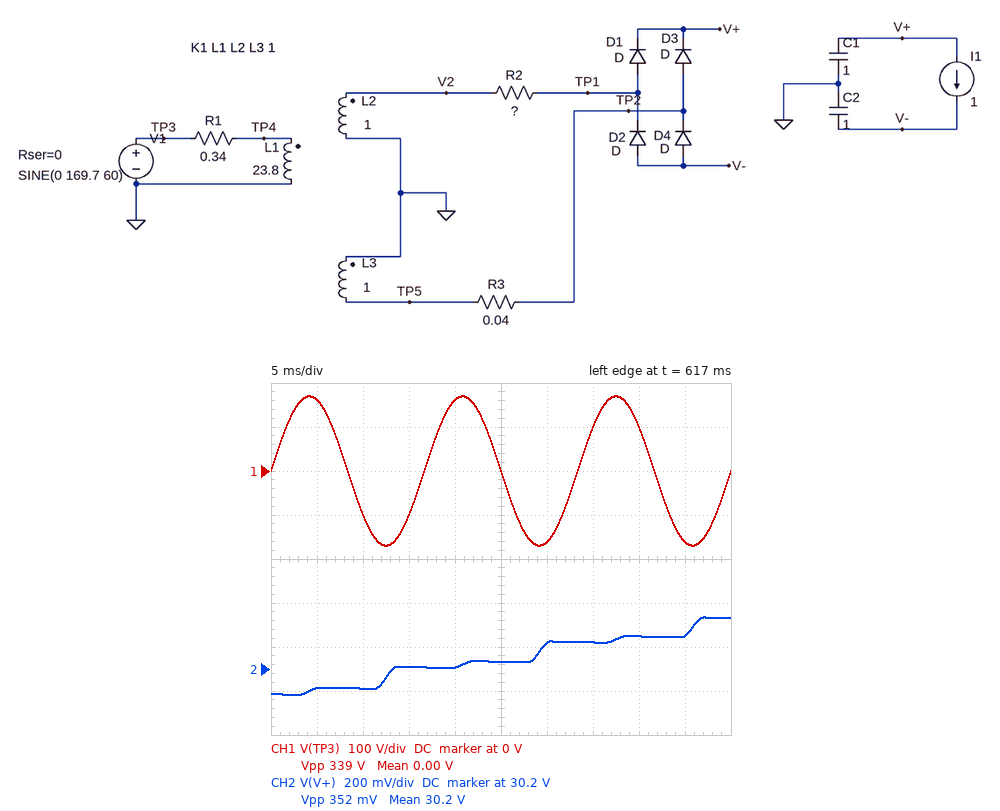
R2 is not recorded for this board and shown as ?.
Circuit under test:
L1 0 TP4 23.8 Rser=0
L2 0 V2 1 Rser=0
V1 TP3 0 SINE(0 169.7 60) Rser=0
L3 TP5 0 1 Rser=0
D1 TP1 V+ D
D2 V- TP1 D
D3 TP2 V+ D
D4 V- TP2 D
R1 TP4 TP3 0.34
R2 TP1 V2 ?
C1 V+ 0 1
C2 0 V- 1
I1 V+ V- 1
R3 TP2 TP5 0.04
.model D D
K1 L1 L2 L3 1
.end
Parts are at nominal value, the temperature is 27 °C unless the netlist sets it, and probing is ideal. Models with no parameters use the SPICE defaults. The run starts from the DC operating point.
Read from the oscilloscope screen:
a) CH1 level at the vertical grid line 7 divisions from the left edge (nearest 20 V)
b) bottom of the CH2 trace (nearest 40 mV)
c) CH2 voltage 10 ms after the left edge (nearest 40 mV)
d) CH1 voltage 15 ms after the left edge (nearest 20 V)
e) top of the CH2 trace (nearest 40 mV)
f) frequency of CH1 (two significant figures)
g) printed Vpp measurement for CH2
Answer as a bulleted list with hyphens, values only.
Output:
- 100 V
- 30.08 V
- 30.12 V
- -100 V
- 30.44 V
- 60 Hz
- 352 mV
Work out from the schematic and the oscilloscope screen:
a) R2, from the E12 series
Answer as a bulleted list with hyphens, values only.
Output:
- 0.12 Ω
